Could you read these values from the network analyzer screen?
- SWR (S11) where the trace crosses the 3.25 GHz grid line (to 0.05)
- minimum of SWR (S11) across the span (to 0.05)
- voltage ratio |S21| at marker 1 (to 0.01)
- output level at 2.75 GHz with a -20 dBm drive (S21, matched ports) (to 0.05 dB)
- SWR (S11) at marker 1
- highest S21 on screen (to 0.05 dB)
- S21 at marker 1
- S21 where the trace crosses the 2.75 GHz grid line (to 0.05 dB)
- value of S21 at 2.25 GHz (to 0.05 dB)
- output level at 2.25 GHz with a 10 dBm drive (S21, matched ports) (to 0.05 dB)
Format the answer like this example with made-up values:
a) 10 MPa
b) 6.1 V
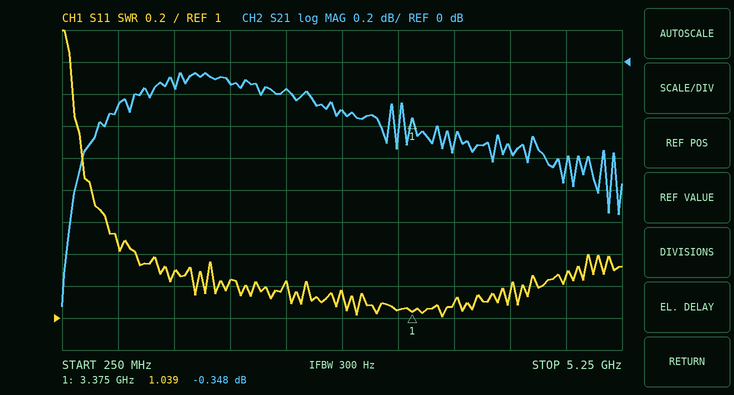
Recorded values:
a) 1.05
b) 1.00
c) 0.96
d) -20.30 dBm
e) 1.039
f) -0.05 dB
g) -0.348 dB
h) -0.30 dB
i) -0.15 dB
j) 9.85 dBm
